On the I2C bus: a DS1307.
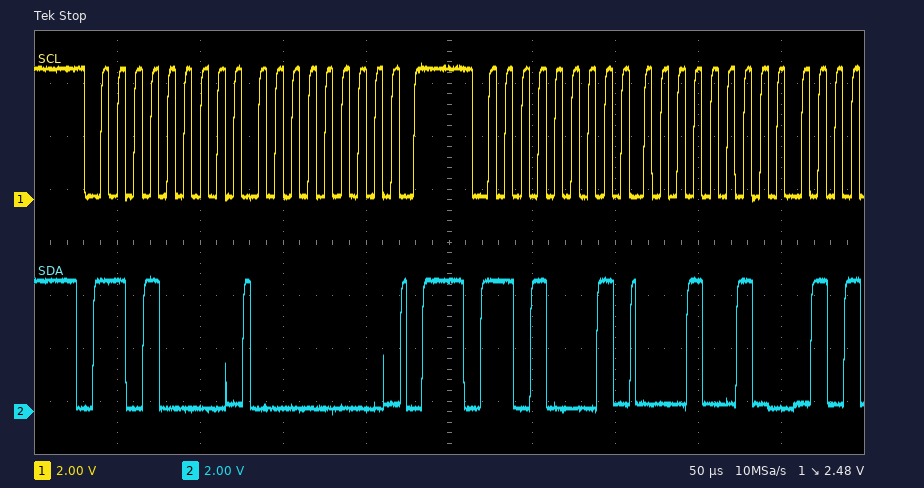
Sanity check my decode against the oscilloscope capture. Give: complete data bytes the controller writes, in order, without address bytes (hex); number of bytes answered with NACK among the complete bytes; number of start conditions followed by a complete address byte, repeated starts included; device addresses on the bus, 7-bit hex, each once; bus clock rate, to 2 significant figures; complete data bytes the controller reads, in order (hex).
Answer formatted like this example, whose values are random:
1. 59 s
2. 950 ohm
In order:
1. 00
2. 0
3. 2
4. 0x68
5. 100 kHz
6. 12
